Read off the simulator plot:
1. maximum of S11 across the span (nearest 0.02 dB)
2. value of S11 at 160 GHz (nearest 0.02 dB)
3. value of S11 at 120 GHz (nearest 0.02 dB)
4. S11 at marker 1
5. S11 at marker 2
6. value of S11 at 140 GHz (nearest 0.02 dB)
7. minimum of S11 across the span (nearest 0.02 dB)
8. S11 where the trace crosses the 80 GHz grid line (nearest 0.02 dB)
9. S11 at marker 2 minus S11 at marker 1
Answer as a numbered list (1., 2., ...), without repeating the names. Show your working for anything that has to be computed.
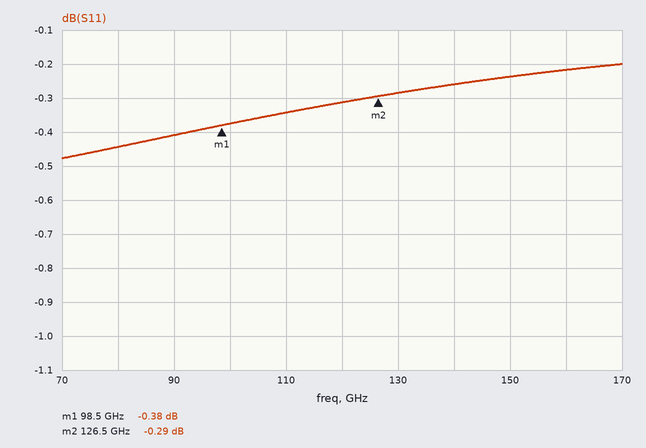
1. -0.20 dB
2. -0.22 dB
3. -0.32 dB
4. -0.38 dB
5. -0.29 dB
6. -0.26 dB
7. -0.48 dB
8. -0.44 dB
9. -0.29 − (-0.38) = 0.09 dB
